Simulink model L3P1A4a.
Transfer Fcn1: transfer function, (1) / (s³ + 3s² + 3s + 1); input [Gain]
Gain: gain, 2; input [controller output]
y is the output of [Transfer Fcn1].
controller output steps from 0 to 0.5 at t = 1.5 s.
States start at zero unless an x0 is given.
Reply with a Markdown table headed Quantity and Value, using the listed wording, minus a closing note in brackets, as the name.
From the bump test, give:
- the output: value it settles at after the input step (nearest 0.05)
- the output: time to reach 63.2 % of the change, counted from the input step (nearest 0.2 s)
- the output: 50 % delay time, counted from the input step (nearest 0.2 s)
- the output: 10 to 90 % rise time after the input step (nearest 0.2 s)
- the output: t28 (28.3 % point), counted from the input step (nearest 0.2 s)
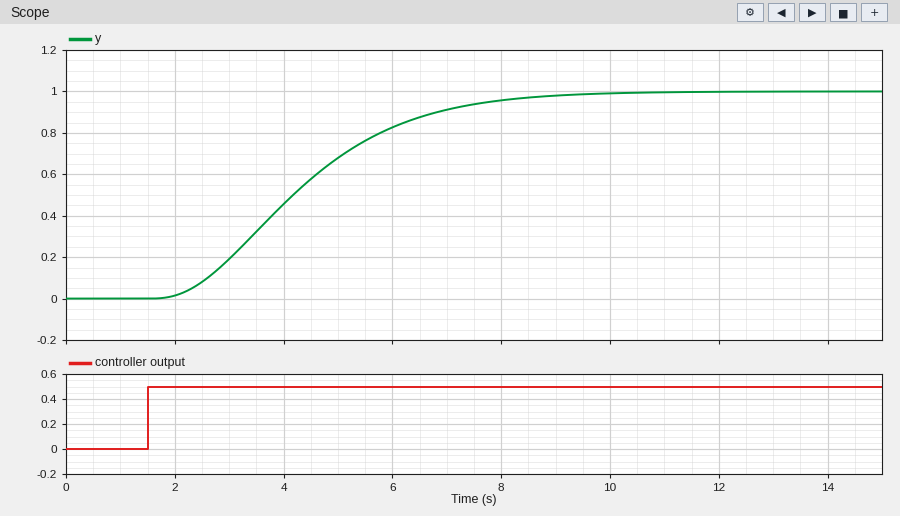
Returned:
| Quantity | Value |
|---|---|
| the output: value it settles at after the input step | 1.00 |
| the output: time to reach 63.2 % of the change, counted from the input step | 3.2 s |
| the output: 50 % delay time, counted from the input step | 2.6 s |
| the output: 10 to 90 % rise time after the input step | 4.2 s |
| the output: t28 (28.3 % point), counted from the input step | 1.8 s |
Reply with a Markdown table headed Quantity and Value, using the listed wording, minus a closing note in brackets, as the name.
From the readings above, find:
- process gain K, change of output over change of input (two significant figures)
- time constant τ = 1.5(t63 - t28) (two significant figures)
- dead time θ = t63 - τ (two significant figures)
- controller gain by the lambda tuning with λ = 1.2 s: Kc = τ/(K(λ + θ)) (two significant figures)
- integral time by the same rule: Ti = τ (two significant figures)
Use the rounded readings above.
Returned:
| Quantity | Value |
|---|---|
| process gain K, change of output over change of input | 2.0 |
| time constant τ = 1.5(t63 - t28) | 2.1 s |
| dead time θ = t63 - τ | 1.1 s |
| controller gain by the lambda tuning with λ = 1.2 s: Kc = τ/(K(λ + θ)) | 0.46 |
| integral time by the same rule: Ti = τ | 2.1 s |
